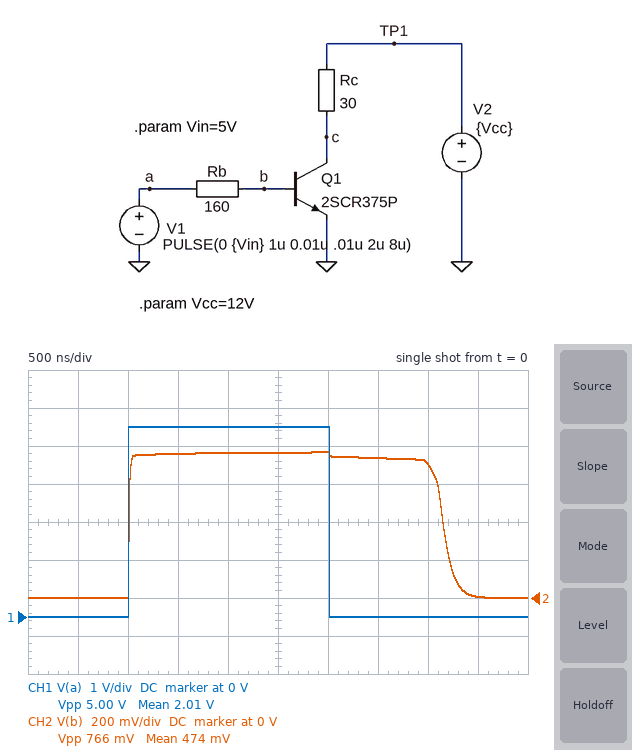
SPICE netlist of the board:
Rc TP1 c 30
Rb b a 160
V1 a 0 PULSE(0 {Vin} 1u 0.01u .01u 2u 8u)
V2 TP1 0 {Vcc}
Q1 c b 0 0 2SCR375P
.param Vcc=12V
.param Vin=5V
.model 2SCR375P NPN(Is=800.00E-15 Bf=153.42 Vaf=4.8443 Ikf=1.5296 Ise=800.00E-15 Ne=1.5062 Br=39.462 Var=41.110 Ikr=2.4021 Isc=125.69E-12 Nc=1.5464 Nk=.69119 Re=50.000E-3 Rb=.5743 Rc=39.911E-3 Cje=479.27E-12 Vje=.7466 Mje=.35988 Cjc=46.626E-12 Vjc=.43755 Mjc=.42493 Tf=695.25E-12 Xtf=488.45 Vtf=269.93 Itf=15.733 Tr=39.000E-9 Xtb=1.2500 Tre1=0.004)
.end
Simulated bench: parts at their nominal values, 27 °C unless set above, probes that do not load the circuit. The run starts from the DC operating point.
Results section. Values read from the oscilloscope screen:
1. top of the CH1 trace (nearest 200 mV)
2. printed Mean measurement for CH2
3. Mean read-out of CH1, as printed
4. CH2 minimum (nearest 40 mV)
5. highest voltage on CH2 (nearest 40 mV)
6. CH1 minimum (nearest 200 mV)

5.0 V
474 mV
2.01 V
0 V
760 mV
0 V
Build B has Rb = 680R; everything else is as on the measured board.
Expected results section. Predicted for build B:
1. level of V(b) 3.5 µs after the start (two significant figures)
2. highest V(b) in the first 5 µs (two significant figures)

610 mV
740 mV
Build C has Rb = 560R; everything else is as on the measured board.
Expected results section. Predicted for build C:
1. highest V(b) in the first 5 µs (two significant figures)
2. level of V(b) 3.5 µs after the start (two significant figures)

740 mV
640 mV
